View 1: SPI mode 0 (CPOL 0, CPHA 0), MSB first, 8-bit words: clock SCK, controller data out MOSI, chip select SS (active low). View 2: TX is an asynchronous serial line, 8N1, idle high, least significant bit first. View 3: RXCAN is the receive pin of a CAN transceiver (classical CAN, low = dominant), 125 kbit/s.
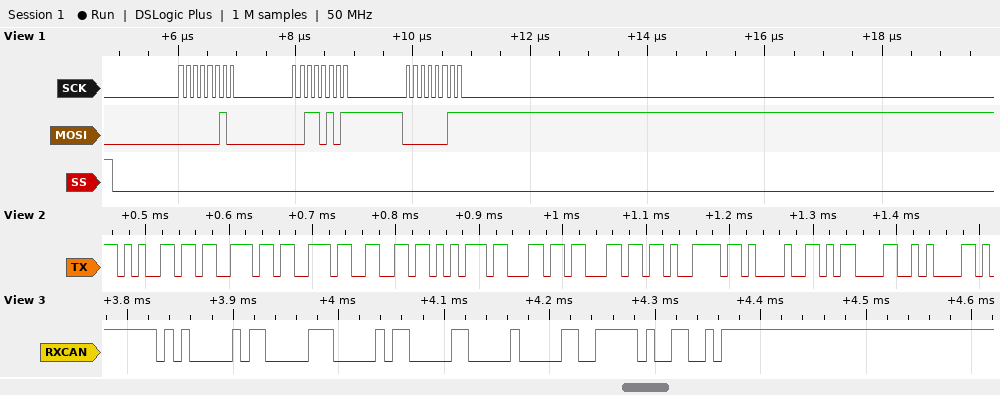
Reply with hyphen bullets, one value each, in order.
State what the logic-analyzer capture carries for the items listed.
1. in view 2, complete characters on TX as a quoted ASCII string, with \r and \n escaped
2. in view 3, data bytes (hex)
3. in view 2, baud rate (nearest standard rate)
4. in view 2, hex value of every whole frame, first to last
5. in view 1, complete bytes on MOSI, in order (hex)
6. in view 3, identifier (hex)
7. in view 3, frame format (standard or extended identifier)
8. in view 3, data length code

- "essfully!\r\n"
- 03 04 00
- 115200 baud
- 65 73 73 66 75 6C 6C 79 21 0D 0A
- 02 35 03
- 0x503
- standard
- 3
